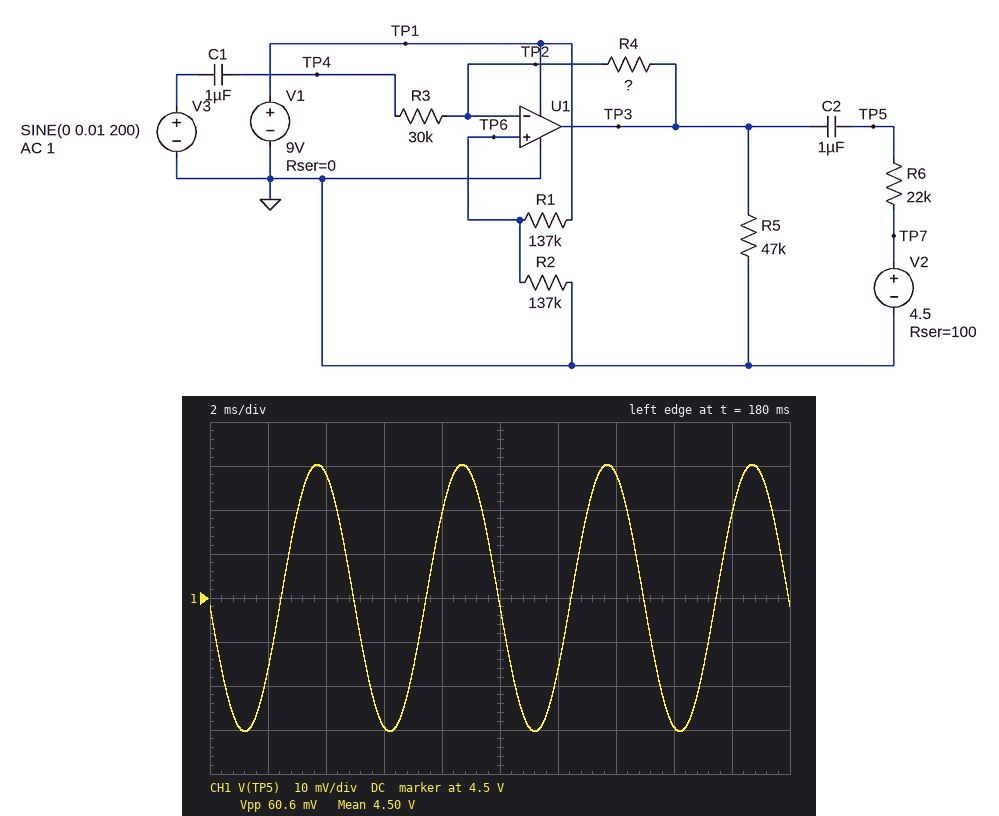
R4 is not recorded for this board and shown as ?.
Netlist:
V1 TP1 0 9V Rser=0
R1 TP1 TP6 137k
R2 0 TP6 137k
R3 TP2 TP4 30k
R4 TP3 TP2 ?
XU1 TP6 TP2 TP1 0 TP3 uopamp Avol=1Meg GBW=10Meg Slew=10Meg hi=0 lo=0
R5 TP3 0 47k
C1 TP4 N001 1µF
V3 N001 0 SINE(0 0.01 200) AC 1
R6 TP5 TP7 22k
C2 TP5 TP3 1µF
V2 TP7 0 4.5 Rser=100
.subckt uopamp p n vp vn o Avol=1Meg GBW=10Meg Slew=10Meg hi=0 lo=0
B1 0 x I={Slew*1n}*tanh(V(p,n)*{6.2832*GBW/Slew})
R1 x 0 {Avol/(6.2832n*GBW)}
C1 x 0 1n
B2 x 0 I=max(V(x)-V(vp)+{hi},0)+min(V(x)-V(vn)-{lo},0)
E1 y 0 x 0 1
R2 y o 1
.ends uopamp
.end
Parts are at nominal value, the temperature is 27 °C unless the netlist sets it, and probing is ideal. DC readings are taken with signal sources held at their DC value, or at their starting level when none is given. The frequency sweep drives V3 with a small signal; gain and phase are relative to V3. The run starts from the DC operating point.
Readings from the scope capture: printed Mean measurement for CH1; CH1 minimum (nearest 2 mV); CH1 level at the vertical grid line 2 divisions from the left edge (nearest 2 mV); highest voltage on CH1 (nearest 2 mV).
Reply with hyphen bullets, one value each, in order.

- 4.50 V
- 4.470 V
- 4.528 V
- 4.530 V
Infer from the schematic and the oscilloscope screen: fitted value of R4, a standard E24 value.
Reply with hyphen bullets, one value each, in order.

- 91 kΩ
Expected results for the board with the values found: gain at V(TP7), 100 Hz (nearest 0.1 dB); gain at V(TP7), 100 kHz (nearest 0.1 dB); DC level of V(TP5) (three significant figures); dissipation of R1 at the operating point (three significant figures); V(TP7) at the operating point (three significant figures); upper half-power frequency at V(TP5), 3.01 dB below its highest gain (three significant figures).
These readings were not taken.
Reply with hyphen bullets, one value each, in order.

- -37.3 dB
- -37.3 dB
- 4.50 V
- 148 µW
- 4.50 V
- 2.48 MHz
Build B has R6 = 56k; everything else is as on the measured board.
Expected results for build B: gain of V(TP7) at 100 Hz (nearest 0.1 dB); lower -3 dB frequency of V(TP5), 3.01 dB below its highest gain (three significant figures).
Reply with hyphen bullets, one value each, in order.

- -45.4 dB
- 6.45 Hz
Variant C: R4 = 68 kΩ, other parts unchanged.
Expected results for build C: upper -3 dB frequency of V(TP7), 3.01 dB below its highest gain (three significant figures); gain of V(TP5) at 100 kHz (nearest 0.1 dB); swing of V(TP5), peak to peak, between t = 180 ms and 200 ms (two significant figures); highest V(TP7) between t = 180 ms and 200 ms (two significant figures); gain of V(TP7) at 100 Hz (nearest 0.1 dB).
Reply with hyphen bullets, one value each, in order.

- 3.06 MHz
- 7.1 dB
- 45 mV
- 4.5 V
- -39.8 dB
